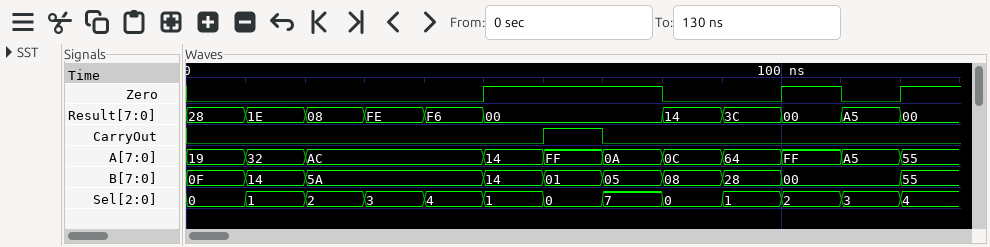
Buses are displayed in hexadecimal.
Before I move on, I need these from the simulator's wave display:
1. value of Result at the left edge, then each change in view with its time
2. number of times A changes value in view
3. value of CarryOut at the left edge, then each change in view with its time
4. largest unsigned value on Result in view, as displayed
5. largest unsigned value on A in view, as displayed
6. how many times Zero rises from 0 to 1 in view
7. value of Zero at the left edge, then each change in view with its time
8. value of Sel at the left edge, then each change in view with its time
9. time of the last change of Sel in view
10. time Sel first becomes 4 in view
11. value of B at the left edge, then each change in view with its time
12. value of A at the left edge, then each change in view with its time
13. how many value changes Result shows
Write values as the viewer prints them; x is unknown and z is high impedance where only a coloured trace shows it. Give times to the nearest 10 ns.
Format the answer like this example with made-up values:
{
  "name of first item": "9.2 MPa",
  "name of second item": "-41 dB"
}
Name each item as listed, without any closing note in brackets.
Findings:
{
  "value of Result at the left edge, then each change in view with its time": "28, 1E at 10 ns, 08 at 20 ns, FE at 30 ns, F6 at 40 ns, 00 at 50 ns, 14 at 80 ns, 3C at 90 ns, 00 at 100 ns, A5 at 110 ns, 00 at 120 ns",
  "number of times A changes value in view": "10",
  "value of CarryOut at the left edge, then each change in view with its time": "0, 1 at 60 ns, 0 at 70 ns",
  "largest unsigned value on Result in view, as displayed": "FE",
  "largest unsigned value on A in view, as displayed": "FF",
  "how many times Zero rises from 0 to 1 in view": "3",
  "value of Zero at the left edge, then each change in view with its time": "0, 1 at 50 ns, 0 at 80 ns, 1 at 100 ns, 0 at 110 ns, 1 at 120 ns",
  "value of Sel at the left edge, then each change in view with its time": "0, 1 at 10 ns, 2 at 20 ns, 3 at 30 ns, 4 at 40 ns, 1 at 50 ns, 0 at 60 ns, 7 at 70 ns, 0 at 80 ns, 1 at 90 ns, 2 at 100 ns, 3 at 110 ns, 4 at 120 ns",
  "time of the last change of Sel in view": "120 ns",
  "time Sel first becomes 4 in view": "40 ns",
  "value of B at the left edge, then each change in view with its time": "0F, 14 at 10 ns, 5A at 20 ns, 14 at 50 ns, 01 at 60 ns, 05 at 70 ns, 08 at 80 ns, 28 at 90 ns, 00 at 100 ns, 55 at 120 ns",
  "value of A at the left edge, then each change in view with its time": "19, 32 at 10 ns, AC at 20 ns, 14 at 50 ns, FF at 60 ns, 0A at 70 ns, 0C at 80 ns, 64 at 90 ns, FF at 100 ns, A5 at 110 ns, 55 at 120 ns",
  "how many value changes Result shows": "10"
}
